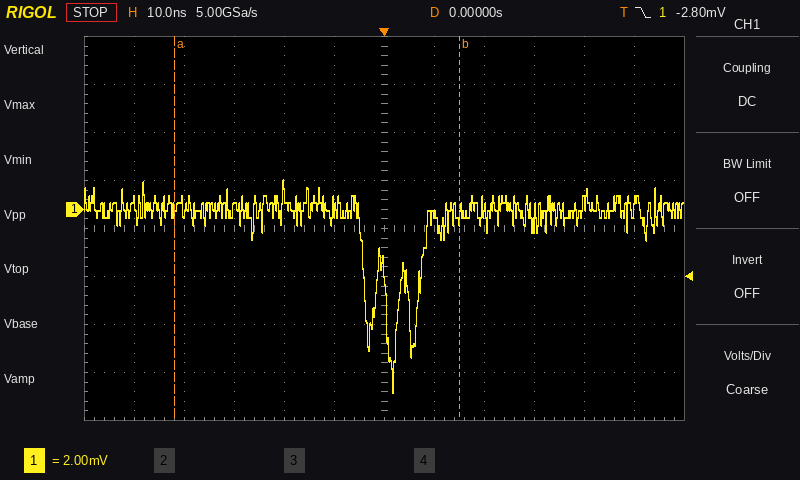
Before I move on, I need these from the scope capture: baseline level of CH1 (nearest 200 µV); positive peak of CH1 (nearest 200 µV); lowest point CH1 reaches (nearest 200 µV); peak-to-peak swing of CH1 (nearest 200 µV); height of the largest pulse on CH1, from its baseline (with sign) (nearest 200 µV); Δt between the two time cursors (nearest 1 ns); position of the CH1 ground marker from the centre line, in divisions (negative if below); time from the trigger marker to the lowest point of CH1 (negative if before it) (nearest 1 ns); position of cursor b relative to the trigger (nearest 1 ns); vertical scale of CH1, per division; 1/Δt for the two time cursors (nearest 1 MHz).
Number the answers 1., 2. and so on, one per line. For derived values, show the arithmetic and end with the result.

1. 0.0 mV
2. 1.2 mV
3. -7.6 mV
4. 1.2 mV − (-7.6 mV) = 8.8 mV
5. -7.6 mV − (0.0 mV) = -7.6 mV
6. 57 ns
7. +0.4 div
8. +2 ns
9. +15 ns
10. 2 mV
11. 1 / 57 ns ≈ 18 MHz
